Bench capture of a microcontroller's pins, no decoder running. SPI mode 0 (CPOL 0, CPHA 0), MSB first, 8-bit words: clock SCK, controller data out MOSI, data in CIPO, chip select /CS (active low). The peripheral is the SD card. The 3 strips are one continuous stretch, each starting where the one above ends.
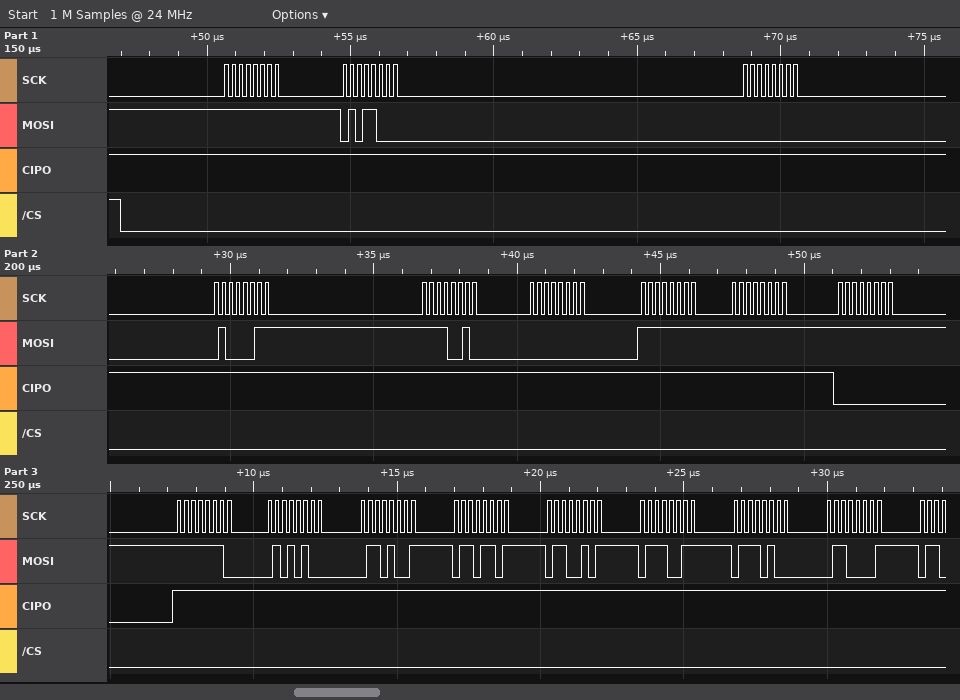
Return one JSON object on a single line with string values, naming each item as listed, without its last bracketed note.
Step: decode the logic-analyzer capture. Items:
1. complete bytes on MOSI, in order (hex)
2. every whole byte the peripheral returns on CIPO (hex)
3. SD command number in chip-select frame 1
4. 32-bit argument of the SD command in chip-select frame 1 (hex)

{"complete bytes on MOSI, in order": "FF 58 00 43 F2 00 FF FF FF FE 54 69 6D 65 73 74 61", "every whole byte the peripheral returns on CIPO": "FF FF FF FF FF FF FF FF 00 FF FF FF FF FF FF FF FF", "SD command number in chip-select frame 1": "CMD24", "32-bit argument of the SD command in chip-select frame 1": "0x0043F200"}
